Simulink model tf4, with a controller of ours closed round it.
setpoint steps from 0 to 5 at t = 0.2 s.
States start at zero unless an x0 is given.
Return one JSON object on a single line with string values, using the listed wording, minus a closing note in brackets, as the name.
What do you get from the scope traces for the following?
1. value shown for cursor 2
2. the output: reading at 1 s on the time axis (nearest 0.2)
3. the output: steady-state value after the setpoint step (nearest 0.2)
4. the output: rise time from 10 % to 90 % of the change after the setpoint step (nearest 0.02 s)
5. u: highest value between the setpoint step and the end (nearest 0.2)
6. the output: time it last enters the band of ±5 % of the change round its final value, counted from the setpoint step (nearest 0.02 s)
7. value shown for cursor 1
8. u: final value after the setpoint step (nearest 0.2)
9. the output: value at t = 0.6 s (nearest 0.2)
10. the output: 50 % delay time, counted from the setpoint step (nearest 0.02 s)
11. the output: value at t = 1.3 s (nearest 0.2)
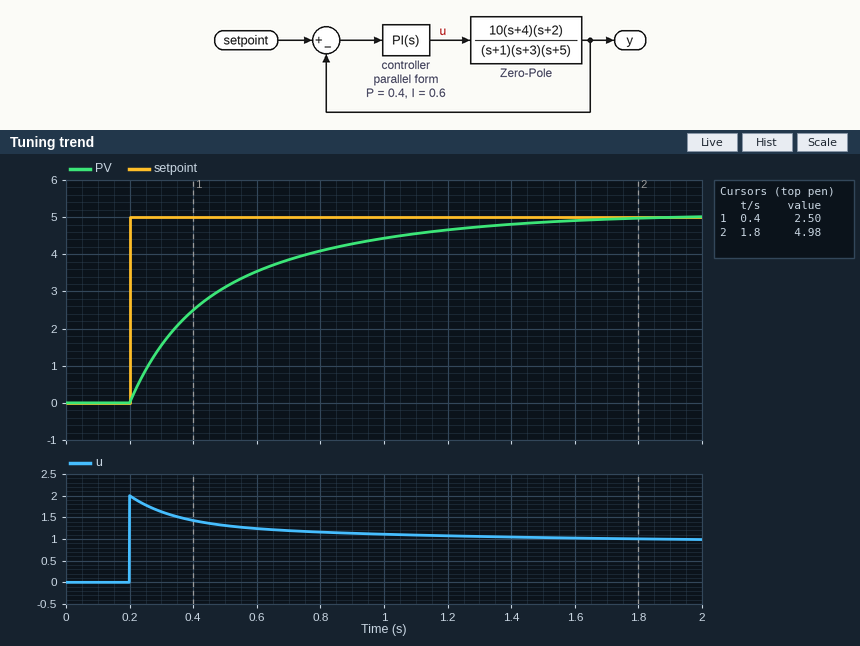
{"value shown for cursor 2": "4.98", "the output: reading at 1 s on the time axis": "4.4", "the output: steady-state value after the setpoint step": "5.0", "the output: rise time from 10 % to 90 % of the change after the setpoint step": "0.82 s", "u: highest value between the setpoint step and the end": "2.0", "the output: time it last enters the band of ±5 % of the change round its final value, counted from the setpoint step": "1.12 s", "value shown for cursor 1": "2.50", "u: final value after the setpoint step": "1.0", "the output: value at t = 0.6 s": "3.6", "the output: 50 % delay time, counted from the setpoint step": "0.20 s", "the output: value at t = 1.3 s": "4.8"}
